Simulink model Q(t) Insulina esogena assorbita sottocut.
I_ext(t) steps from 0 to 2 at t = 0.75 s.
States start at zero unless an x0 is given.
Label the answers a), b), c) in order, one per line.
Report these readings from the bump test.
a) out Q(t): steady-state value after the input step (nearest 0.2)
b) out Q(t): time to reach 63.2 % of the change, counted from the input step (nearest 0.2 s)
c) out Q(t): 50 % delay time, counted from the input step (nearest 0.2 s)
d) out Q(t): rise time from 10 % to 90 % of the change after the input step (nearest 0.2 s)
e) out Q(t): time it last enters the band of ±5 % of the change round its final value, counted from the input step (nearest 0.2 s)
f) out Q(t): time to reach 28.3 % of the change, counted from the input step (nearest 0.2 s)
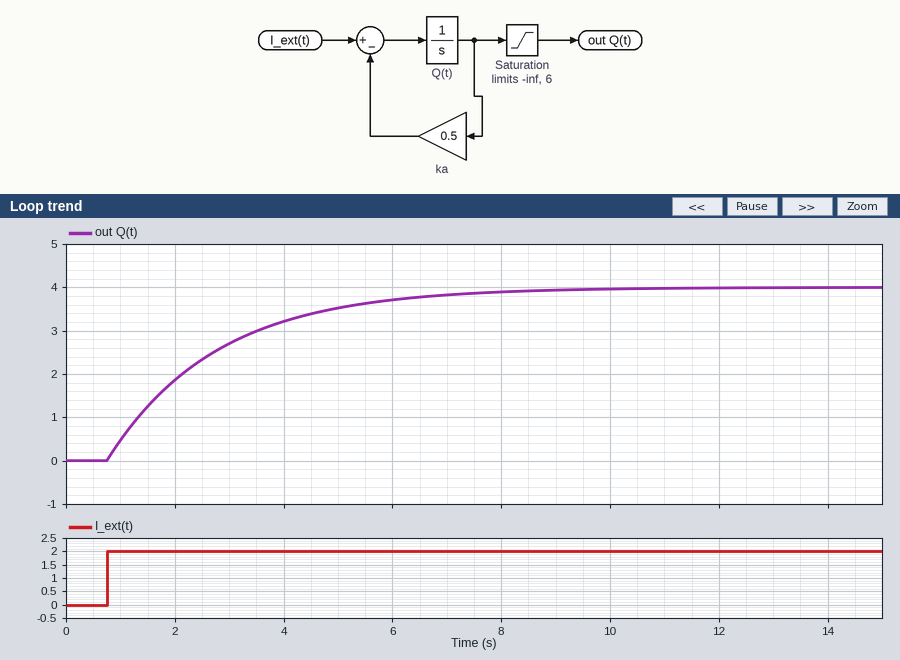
a) 4.0
b) 2.0 s
c) 1.4 s
d) 4.4 s
e) 6.0 s
f) 0.6 s
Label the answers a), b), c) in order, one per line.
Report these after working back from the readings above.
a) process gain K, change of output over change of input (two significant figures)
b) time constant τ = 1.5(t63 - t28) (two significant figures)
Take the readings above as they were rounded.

a) 2.0
b) 2.1 s
